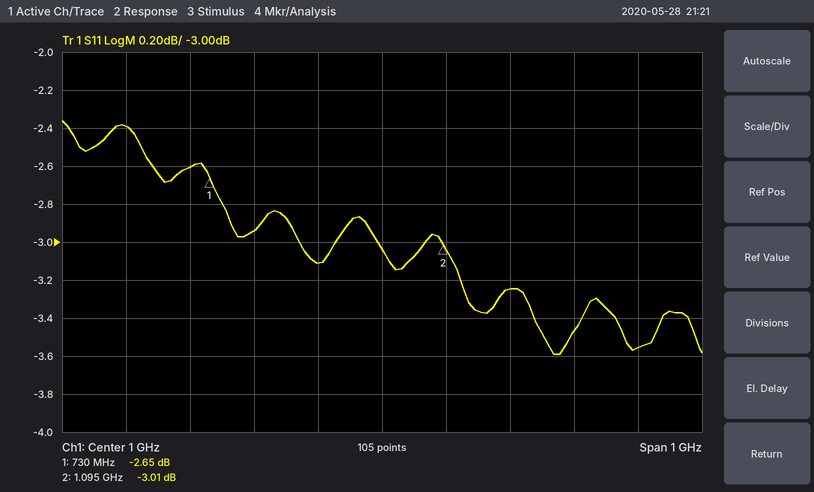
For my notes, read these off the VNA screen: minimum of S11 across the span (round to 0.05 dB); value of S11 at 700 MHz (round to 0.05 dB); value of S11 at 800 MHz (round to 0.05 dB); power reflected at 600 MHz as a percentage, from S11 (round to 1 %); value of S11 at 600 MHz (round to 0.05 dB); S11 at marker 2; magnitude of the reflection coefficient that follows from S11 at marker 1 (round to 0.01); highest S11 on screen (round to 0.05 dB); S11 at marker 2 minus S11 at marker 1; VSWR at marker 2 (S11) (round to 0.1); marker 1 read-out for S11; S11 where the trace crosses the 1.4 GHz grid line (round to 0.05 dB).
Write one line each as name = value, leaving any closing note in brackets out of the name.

minimum of S11 across the span = -3.60 dB
value of S11 at 700 MHz = -2.60 dB
value of S11 at 800 MHz = -2.95 dB
power reflected at 600 MHz as a percentage, from S11 = 58 %
value of S11 at 600 MHz = -2.40 dB
S11 at marker 2 = -3.01 dB
magnitude of the reflection coefficient that follows from S11 at marker 1 = 0.74
highest S11 on screen = -2.35 dB
S11 at marker 2 minus S11 at marker 1 = -0.36 dB
VSWR at marker 2 (S11) = 5.8
marker 1 read-out for S11 = -2.65 dB
S11 where the trace crosses the 1.4 GHz grid line = -3.55 dB
